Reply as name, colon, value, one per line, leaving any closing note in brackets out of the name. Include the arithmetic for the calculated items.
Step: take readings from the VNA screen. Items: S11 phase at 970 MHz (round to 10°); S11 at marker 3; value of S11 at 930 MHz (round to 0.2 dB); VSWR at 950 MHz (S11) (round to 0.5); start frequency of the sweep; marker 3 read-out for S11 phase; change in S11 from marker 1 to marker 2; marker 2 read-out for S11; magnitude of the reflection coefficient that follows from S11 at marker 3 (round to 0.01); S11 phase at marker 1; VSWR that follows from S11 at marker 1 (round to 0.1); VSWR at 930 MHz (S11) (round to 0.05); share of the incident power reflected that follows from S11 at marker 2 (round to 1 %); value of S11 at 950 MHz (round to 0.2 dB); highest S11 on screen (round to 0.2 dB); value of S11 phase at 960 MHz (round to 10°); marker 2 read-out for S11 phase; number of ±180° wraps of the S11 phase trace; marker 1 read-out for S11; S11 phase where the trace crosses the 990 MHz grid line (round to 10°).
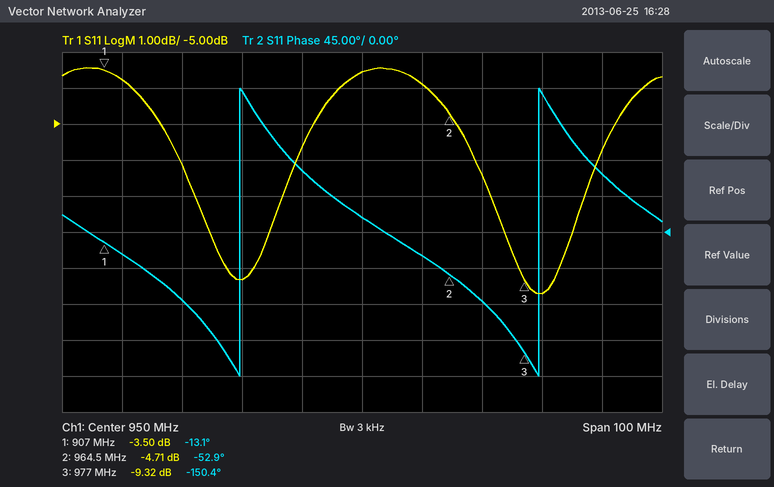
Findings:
S11 phase at 970 MHz: -90°
S11 at marker 3: -9.32 dB
value of S11 at 930 MHz: -9.4 dB
VSWR at 950 MHz (S11): |Γ| = 10^(-3.6/20) = 0.6607; VSWR = (1 + 0.6607)/(1 − 0.6607) ≈ 4.89, so 5.0 to the nearest 0.5
start frequency of the sweep: 900 MHz
marker 3 read-out for S11 phase: -150.4°
change in S11 from marker 1 to marker 2: -4.71 − (-3.5) = -1.21 dB
marker 2 read-out for S11: -4.71 dB
magnitude of the reflection coefficient that follows from S11 at marker 3: 10^(-9.32/20) ≈ 0.34
S11 phase at marker 1: -13.1°
VSWR that follows from S11 at marker 1: (1 + 0.6683)/(1 − 0.6683) ≈ 5.0
VSWR at 930 MHz (S11): |Γ| = 10^(-9.4/20) = 0.3388; VSWR = (1 + 0.3388)/(1 − 0.3388) ≈ 2.03, so 2.05 to the nearest 0.05
share of the incident power reflected that follows from S11 at marker 2: 10^(-4.71/10) ≈ 34 %
value of S11 at 950 MHz: -3.6 dB
highest S11 on screen: -3.4 dB
value of S11 phase at 960 MHz: -30°
marker 2 read-out for S11 phase: -52.9°
number of ±180° wraps of the S11 phase trace: 2
marker 1 read-out for S11: -3.50 dB
S11 phase where the trace crosses the 990 MHz grid line: 70°
